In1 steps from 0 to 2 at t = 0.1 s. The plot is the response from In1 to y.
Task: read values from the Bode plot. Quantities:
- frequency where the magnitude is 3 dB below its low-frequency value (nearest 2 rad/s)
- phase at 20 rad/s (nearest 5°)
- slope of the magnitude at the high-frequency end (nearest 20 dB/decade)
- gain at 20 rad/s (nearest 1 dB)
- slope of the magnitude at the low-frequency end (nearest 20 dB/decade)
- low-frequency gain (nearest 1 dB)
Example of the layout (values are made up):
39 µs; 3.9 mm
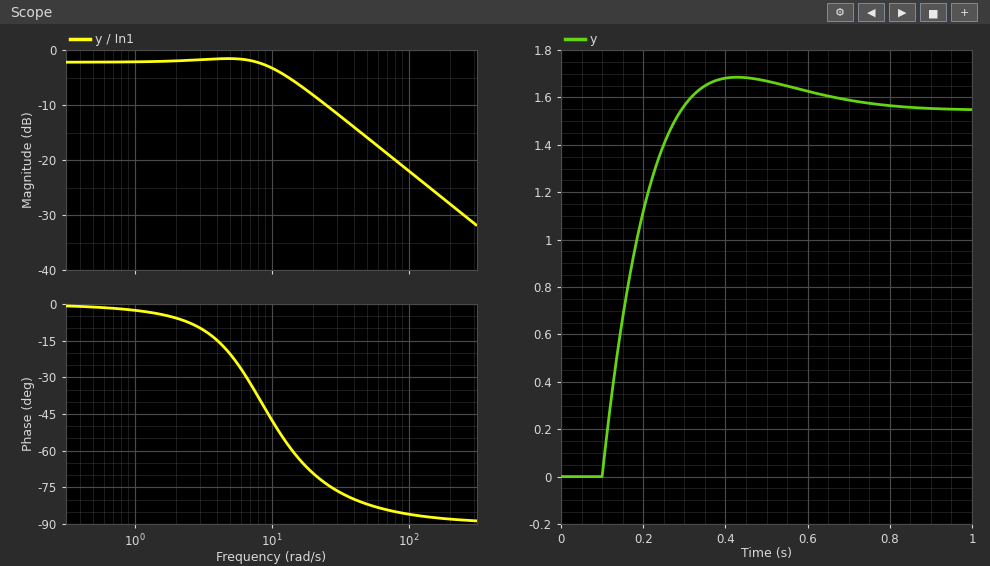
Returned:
14 rad/s; -70°; -20 dB/decade; -8 dB; 0 dB/decade; -2 dB
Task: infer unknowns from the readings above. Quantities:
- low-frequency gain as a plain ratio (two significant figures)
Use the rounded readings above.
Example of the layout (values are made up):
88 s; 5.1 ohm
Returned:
0.79
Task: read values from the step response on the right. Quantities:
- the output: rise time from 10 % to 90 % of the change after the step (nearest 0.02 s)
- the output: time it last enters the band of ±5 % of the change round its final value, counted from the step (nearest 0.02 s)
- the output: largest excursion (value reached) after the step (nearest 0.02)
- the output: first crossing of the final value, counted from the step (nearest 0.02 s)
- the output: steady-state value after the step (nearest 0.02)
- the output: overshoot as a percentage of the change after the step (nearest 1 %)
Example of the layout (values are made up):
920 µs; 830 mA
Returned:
0.14 s; 0.50 s; 1.68; 0.20 s; 1.54; 9 %
